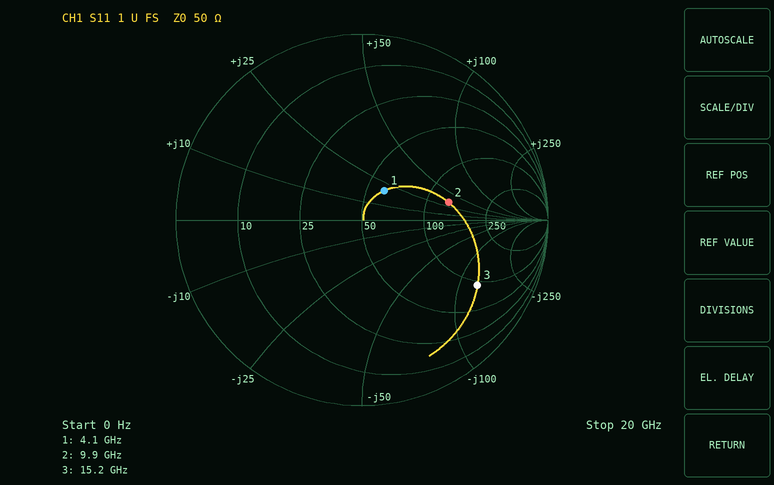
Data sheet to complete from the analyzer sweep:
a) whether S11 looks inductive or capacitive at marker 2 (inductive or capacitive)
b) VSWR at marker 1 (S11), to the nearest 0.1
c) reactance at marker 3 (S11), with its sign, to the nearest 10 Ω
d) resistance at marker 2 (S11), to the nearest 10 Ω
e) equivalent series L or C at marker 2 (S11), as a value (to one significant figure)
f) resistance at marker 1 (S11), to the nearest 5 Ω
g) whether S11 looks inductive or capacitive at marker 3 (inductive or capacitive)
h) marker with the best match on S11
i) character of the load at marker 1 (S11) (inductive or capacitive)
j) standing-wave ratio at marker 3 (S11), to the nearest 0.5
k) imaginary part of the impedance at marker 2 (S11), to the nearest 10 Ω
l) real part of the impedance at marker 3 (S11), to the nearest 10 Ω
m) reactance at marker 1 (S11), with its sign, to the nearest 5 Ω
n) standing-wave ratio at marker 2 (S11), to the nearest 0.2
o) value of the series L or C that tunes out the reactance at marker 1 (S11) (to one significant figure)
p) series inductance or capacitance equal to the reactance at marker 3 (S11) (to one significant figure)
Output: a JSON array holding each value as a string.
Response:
["inductive", "1.5", "-130 Ω", "130 Ω", "500 pH", "60 Ω", "capacitive", "marker 1", "inductive", "6.0", "+30 Ω", "90 Ω", "+20 Ω", "2.8", "2 pF", "80 fF"]
